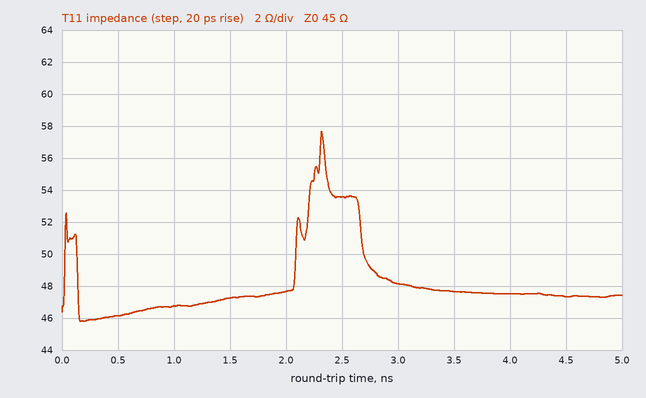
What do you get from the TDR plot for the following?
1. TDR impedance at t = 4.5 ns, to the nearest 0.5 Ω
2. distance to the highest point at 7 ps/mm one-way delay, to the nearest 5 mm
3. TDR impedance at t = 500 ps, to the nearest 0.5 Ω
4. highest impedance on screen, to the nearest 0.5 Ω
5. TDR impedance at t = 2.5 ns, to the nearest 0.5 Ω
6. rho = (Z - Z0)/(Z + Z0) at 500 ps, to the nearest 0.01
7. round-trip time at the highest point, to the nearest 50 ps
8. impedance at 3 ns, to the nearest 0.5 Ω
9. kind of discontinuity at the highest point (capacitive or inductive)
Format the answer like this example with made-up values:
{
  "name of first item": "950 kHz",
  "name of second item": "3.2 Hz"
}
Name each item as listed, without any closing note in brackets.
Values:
{
  "TDR impedance at t = 4.5 ns, to the nearest 0.5 Ω": "47.5 Ω",
  "distance to the highest point at 7 ps/mm one-way delay, to the nearest 5 mm": "165 mm",
  "TDR impedance at t = 500 ps, to the nearest 0.5 Ω": "46.0 Ω",
  "highest impedance on screen, to the nearest 0.5 Ω": "57.5 Ω",
  "TDR impedance at t = 2.5 ns, to the nearest 0.5 Ω": "53.5 Ω",
  "rho = (Z - Z0)/(Z + Z0) at 500 ps, to the nearest 0.01": "+0.01",
  "round-trip time at the highest point, to the nearest 50 ps": "2.30 ns",
  "impedance at 3 ns, to the nearest 0.5 Ω": "48.0 Ω",
  "kind of discontinuity at the highest point": "inductive"
}
